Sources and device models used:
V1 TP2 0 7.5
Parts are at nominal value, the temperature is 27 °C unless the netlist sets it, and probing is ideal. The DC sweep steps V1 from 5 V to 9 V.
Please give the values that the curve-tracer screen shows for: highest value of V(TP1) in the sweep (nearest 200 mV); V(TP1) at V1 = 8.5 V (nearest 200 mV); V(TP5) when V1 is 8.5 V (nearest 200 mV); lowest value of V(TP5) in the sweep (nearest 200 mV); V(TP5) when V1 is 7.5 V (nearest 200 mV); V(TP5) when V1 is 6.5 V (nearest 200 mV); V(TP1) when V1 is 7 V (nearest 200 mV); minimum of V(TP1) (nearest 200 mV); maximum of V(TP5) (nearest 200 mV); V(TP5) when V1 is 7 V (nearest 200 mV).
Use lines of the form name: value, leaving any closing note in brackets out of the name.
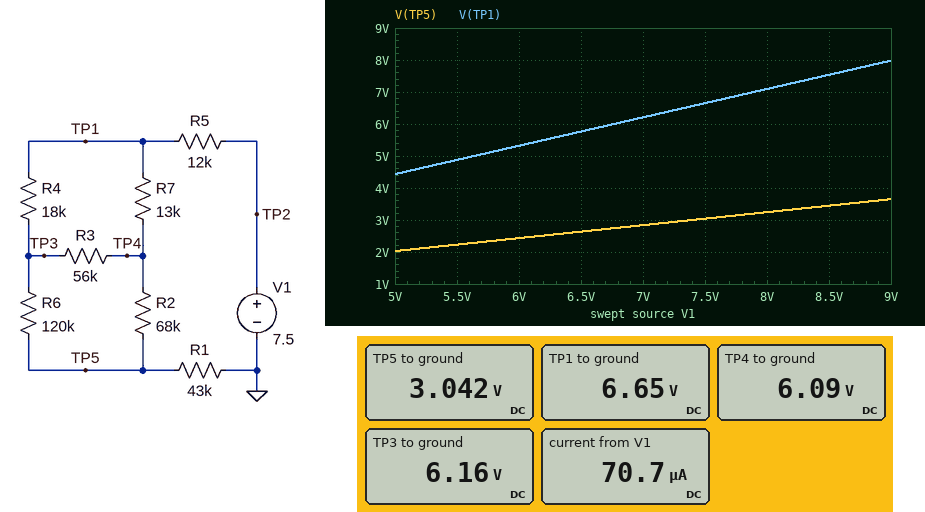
highest value of V(TP1) in the sweep: 8.0 V
V(TP1) at V1 = 8.5 V: 7.6 V
V(TP5) when V1 is 8.5 V: 3.4 V
lowest value of V(TP5) in the sweep: 2.0 V
V(TP5) when V1 is 7.5 V: 3.0 V
V(TP5) when V1 is 6.5 V: 2.6 V
V(TP1) when V1 is 7 V: 6.2 V
minimum of V(TP1): 4.4 V
maximum of V(TP5): 3.6 V
V(TP5) when V1 is 7 V: 2.8 V
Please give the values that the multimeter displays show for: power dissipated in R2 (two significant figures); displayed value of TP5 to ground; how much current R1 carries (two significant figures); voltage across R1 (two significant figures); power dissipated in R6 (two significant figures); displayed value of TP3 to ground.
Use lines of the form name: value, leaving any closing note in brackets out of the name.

power dissipated in R2: 140 µW
displayed value of TP5 to ground: 3.042 V
how much current R1 carries: 71 µA
voltage across R1: 3.0 V
power dissipated in R6: 81 µW
displayed value of TP3 to ground: 6.16 V
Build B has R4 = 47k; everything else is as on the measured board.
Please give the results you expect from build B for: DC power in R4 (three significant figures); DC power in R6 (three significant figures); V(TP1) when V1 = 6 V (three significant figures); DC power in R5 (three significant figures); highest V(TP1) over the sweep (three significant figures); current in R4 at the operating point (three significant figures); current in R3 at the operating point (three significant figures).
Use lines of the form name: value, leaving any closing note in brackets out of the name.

DC power in R4: 17.1 µW
DC power in R6: 66.4 µW
V(TP1) when V1 = 6 V: 5.34 V
DC power in R5: 56.7 µW
highest V(TP1) over the sweep: 8.01 V
current in R4 at the operating point: 19.1 µA
current in R3 at the operating point: 4.47 µA
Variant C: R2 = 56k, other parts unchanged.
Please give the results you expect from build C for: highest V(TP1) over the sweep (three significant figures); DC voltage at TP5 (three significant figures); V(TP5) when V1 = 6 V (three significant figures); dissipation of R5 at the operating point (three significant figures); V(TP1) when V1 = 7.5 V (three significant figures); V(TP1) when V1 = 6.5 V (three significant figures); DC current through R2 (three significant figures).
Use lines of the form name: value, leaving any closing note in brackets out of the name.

highest V(TP1) over the sweep: 7.93 V
DC voltage at TP5: 3.20 V
V(TP5) when V1 = 6 V: 2.56 V
dissipation of R5 at the operating point: 66.3 µW
V(TP1) when V1 = 7.5 V: 6.61 V
V(TP1) when V1 = 6.5 V: 5.73 V
DC current through R2: 49.9 µA
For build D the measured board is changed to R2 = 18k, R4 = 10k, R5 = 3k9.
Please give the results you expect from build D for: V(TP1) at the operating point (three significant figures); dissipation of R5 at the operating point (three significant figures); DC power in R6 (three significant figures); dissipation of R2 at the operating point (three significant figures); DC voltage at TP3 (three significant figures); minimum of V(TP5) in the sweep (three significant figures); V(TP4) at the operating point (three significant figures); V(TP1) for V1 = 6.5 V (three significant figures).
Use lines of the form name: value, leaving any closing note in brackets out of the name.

V(TP1) at the operating point: 7.09 V
dissipation of R5 at the operating point: 43.6 µW
DC power in R6: 41.7 µW
dissipation of R2 at the operating point: 136 µW
DC voltage at TP3: 6.78 V
minimum of V(TP5) in the sweep: 3.03 V
V(TP4) at the operating point: 6.11 V
V(TP1) for V1 = 6.5 V: 6.14 V
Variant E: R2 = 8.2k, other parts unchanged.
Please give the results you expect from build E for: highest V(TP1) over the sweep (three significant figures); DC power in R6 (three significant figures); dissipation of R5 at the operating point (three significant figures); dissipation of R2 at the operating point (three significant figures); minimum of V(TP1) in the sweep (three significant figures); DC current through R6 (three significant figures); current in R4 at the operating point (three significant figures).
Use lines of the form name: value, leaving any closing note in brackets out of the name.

highest V(TP1) over the sweep: 7.51 V
DC power in R6: 16.1 µW
dissipation of R5 at the operating point: 129 µW
dissipation of R2 at the operating point: 69.4 µW
minimum of V(TP1) in the sweep: 4.17 V
DC current through R6: 11.6 µA
current in R4 at the operating point: 22.9 µA
